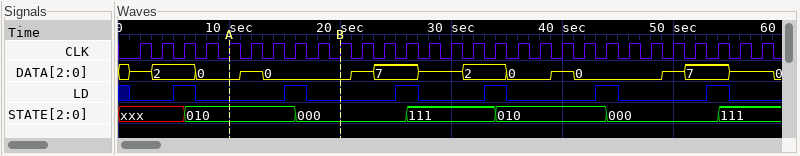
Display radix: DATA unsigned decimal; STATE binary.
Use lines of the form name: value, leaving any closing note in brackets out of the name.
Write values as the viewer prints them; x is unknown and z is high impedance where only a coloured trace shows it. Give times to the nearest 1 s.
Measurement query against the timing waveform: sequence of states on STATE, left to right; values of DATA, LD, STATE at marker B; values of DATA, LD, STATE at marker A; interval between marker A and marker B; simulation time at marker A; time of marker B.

sequence of states on STATE, left to right: xxx, 010, 000, 111, 010, 000, 111
values of DATA, LD, STATE at marker B: DATA=0, LD=0, STATE=000
values of DATA, LD, STATE at marker A: DATA=0, LD=0, STATE=010
interval between marker A and marker B: 10 s
simulation time at marker A: 10 s
time of marker B: 20 s
